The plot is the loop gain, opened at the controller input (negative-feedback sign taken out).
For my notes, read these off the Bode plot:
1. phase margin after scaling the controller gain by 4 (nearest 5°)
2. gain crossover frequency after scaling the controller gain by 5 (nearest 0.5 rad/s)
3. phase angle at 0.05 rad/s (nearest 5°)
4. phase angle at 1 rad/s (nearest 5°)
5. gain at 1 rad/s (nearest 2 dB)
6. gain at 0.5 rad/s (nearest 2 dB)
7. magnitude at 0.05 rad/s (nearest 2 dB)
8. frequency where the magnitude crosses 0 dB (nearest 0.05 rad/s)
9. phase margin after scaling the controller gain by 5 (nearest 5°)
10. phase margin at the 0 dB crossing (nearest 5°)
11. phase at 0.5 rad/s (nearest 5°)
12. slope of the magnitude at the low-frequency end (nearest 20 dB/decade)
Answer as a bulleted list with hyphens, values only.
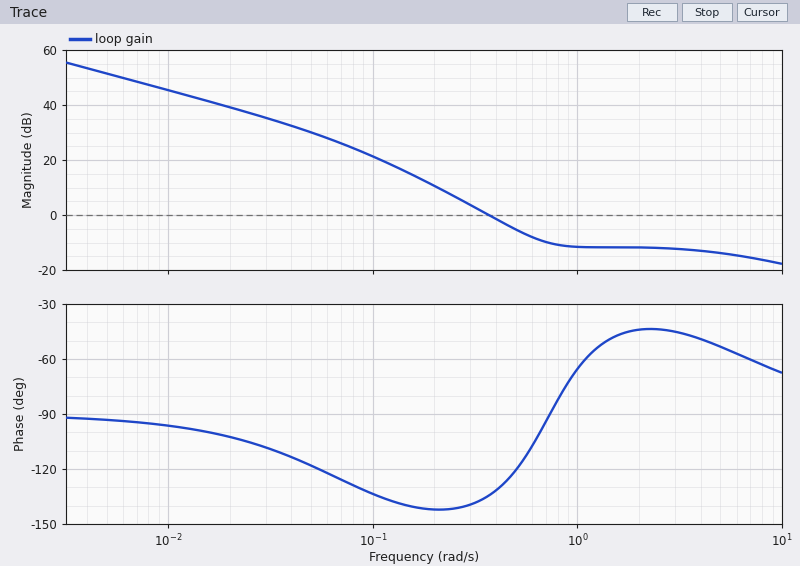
- 135°
- 5.0 rad/s
- -120°
- -65°
- -12 dB
- -6 dB
- 30 dB
- 0.35 rad/s
- 125°
- 45°
- -120°
- -20 dB/decade
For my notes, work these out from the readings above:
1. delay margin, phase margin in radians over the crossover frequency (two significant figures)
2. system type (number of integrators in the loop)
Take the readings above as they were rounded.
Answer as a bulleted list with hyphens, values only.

- 2.2 s
- 1
